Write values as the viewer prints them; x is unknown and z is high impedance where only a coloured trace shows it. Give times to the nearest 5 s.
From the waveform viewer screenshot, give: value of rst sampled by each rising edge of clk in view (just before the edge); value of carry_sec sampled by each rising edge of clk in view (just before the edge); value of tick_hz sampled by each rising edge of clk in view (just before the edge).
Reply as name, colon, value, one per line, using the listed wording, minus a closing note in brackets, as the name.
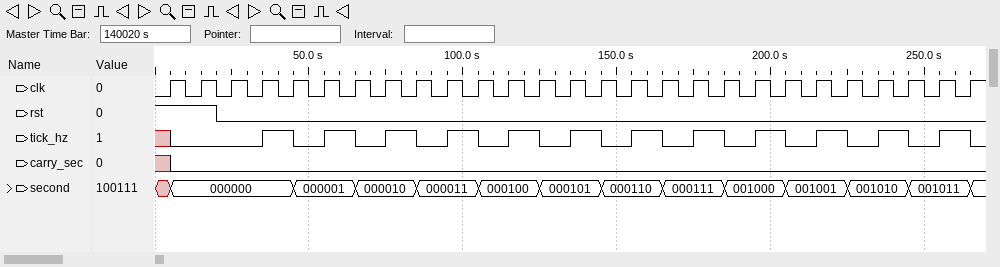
value of rst sampled by each rising edge of clk in view: 1 1 0 0 0 0 0 0 0 0 0 0 0 0 0 0 0 0 0 0 0 0 0 0 0 0 0
value of carry_sec sampled by each rising edge of clk in view: x 0 0 0 0 0 0 0 0 0 0 0 0 0 0 0 0 0 0 0 0 0 0 0 0 0 0
value of tick_hz sampled by each rising edge of clk in view: x 0 0 0 1 0 1 0 1 0 1 0 1 0 1 0 1 0 1 0 1 0 1 0 1 0 1
